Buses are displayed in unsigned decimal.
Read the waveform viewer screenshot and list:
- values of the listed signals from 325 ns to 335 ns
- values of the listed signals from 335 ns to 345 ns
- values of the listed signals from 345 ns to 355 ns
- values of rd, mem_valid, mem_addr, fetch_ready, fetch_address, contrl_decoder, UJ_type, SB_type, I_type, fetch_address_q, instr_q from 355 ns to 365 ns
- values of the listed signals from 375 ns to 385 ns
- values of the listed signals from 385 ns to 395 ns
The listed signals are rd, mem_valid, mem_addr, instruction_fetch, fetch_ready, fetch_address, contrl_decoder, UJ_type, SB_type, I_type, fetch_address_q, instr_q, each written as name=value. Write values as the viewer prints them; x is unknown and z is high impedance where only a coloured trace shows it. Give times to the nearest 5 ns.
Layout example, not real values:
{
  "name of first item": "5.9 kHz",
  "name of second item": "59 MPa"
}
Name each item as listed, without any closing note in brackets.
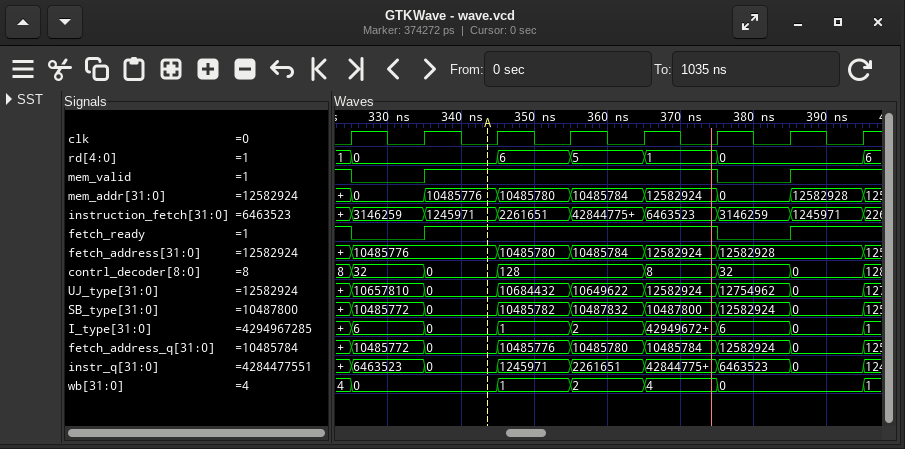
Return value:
{
  "values of the listed signals from 325 ns to 335 ns": "rd=0, mem_valid=0, mem_addr=0, instruction_fetch=3146259, fetch_ready=0, fetch_address=10485776, contrl_decoder=32, UJ_type=10657810, SB_type=10485772, I_type=6, fetch_address_q=10485772, instr_q=6463523",
  "values of the listed signals from 335 ns to 345 ns": "rd=0, mem_valid=1, mem_addr=10485776, instruction_fetch=1245971, fetch_ready=1, fetch_address=10485776, contrl_decoder=0, UJ_type=0, SB_type=0, I_type=0, fetch_address_q=0, instr_q=0",
  "values of the listed signals from 345 ns to 355 ns": "rd=6, mem_valid=1, mem_addr=10485780, instruction_fetch=2261651, fetch_ready=1, fetch_address=10485780, contrl_decoder=128, UJ_type=10684432, SB_type=10485782, I_type=1, fetch_address_q=10485776, instr_q=1245971",
  "values of rd, mem_valid, mem_addr, fetch_ready, fetch_address, contrl_decoder, UJ_type, SB_type, I_type, fetch_address_q, instr_q from 355 ns to 365 ns": "rd=5, mem_valid=1, mem_addr=10485784, fetch_ready=1, fetch_address=10485784, contrl_decoder=128, UJ_type=10649622, SB_type=10487832, I_type=2, fetch_address_q=10485780, instr_q=2261651",
  "values of the listed signals from 375 ns to 385 ns": "rd=0, mem_valid=0, mem_addr=0, instruction_fetch=3146259, fetch_ready=0, fetch_address=12582928, contrl_decoder=32, UJ_type=12754962, SB_type=12582924, I_type=6, fetch_address_q=12582924, instr_q=6463523",
  "values of the listed signals from 385 ns to 395 ns": "rd=0, mem_valid=1, mem_addr=12582928, instruction_fetch=1245971, fetch_ready=1, fetch_address=12582928, contrl_decoder=0, UJ_type=0, SB_type=0, I_type=0, fetch_address_q=0, instr_q=0"
}
